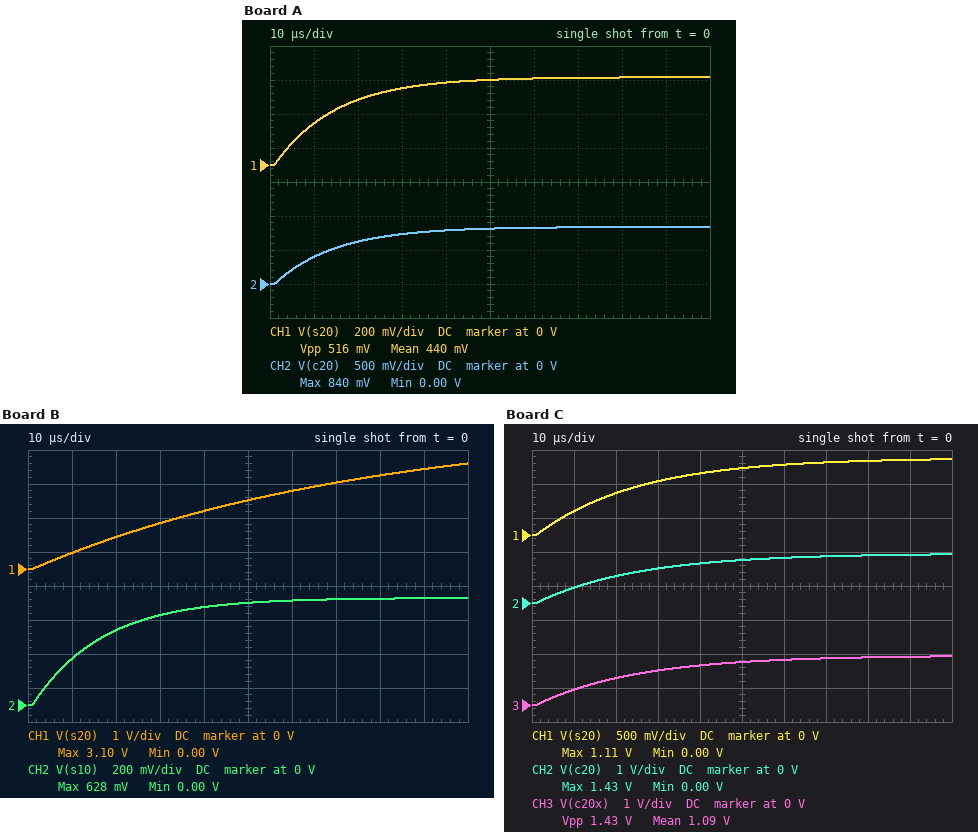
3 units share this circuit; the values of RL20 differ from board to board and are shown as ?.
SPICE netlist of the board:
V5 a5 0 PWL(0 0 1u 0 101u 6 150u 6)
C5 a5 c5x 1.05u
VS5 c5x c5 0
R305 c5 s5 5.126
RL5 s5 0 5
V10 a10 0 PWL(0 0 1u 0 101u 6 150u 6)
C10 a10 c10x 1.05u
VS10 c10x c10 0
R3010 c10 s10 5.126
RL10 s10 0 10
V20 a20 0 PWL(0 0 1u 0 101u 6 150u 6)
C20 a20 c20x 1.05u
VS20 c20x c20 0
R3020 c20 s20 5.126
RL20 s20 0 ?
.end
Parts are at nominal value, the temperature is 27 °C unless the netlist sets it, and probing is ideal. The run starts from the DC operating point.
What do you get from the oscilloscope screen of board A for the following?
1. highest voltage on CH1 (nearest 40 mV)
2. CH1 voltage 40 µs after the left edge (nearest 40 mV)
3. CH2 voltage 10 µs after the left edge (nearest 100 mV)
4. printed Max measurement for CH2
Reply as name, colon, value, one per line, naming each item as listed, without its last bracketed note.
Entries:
highest voltage on CH1: 520 mV
CH1 voltage 40 µs after the left edge: 480 mV
CH2 voltage 10 µs after the left edge: 400 mV
printed Max measurement for CH2: 840 mV
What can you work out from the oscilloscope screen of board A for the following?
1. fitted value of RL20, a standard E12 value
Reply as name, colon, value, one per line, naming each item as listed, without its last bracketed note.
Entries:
fitted value of RL20, a standard E12 value: 8.2 Ω
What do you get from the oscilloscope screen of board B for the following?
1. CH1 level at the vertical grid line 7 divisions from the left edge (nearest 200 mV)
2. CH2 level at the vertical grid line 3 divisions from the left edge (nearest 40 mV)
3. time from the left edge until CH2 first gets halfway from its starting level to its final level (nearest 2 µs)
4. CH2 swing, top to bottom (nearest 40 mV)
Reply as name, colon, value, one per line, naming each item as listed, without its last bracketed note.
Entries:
CH1 level at the vertical grid line 7 divisions from the left edge: 2.6 V
CH2 level at the vertical grid line 3 divisions from the left edge: 520 mV
time from the left edge until CH2 first gets halfway from its starting level to its final level: 12 µs
CH2 swing, top to bottom: 640 mV
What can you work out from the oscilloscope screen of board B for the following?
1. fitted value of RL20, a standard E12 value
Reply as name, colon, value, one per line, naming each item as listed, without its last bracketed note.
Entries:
fitted value of RL20, a standard E12 value: 68 Ω
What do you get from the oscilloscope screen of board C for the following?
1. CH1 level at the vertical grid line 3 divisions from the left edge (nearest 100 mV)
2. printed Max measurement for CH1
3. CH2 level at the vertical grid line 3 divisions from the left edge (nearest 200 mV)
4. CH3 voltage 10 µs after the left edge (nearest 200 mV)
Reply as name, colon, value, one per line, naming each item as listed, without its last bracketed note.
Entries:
CH1 level at the vertical grid line 3 divisions from the left edge: 800 mV
printed Max measurement for CH1: 1.11 V
CH2 level at the vertical grid line 3 divisions from the left edge: 1.0 V
CH3 voltage 10 µs after the left edge: 400 mV
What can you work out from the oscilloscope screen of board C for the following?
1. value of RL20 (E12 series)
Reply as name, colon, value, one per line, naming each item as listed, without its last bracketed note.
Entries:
value of RL20: 18 Ω
